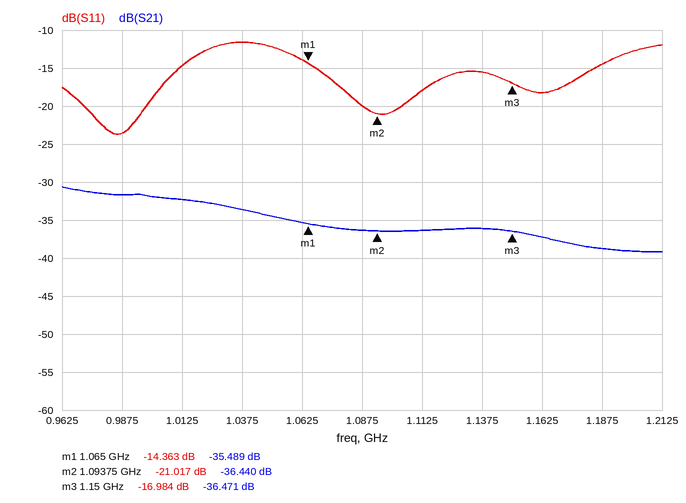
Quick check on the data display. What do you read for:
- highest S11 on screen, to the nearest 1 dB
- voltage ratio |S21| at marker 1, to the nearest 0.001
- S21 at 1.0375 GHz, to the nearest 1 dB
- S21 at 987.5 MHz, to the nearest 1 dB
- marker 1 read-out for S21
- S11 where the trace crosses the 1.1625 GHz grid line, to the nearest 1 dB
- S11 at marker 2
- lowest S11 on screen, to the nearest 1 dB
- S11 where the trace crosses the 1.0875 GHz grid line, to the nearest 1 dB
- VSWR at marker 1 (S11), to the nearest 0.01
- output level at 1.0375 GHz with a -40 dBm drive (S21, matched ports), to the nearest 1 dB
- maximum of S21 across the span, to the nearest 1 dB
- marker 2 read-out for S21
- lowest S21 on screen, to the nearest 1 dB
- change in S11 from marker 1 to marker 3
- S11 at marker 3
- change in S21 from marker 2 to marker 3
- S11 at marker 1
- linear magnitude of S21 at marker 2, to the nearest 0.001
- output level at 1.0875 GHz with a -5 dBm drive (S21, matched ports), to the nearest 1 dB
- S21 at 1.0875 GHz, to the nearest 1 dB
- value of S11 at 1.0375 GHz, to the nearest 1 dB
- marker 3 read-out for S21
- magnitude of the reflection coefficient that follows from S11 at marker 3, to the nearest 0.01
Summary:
-12 dB
0.017
-34 dB
-32 dB
-35.489 dB
-18 dB
-21.017 dB
-24 dB
-20 dB
1.47
-74 dBm
-31 dB
-36.440 dB
-39 dB
-2.621 dB
-16.984 dB
-0.031 dB
-14.363 dB
0.015
-41 dBm
-36 dB
-12 dB
-36.471 dB
0.14
